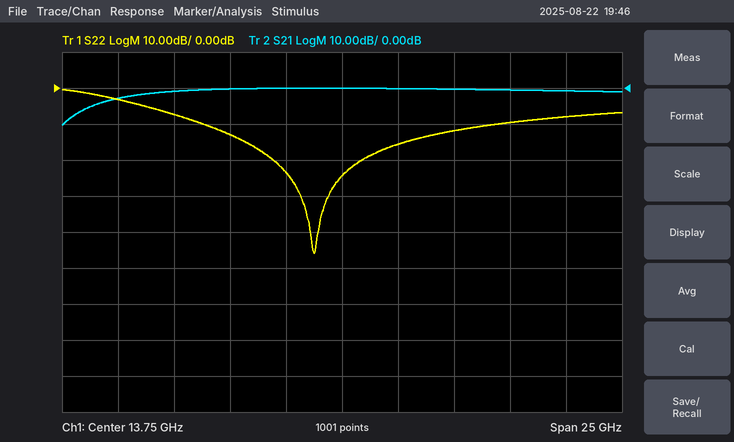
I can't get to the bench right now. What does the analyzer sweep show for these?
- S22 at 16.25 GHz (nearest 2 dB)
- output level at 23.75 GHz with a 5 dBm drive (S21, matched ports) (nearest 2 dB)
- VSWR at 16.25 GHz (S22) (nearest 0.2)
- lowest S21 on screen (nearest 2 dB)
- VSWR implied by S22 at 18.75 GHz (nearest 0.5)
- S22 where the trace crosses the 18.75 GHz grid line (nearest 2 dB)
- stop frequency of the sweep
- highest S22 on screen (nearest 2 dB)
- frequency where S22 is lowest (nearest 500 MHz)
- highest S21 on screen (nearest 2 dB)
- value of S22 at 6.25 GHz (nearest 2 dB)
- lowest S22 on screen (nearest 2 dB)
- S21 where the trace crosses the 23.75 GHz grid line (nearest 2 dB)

-16 dB
4 dBm
1.4
-10 dB
1.5
-12 dB
26.25 GHz
0 dB
12.5 GHz
0 dB
-8 dB
-46 dB
0 dB
